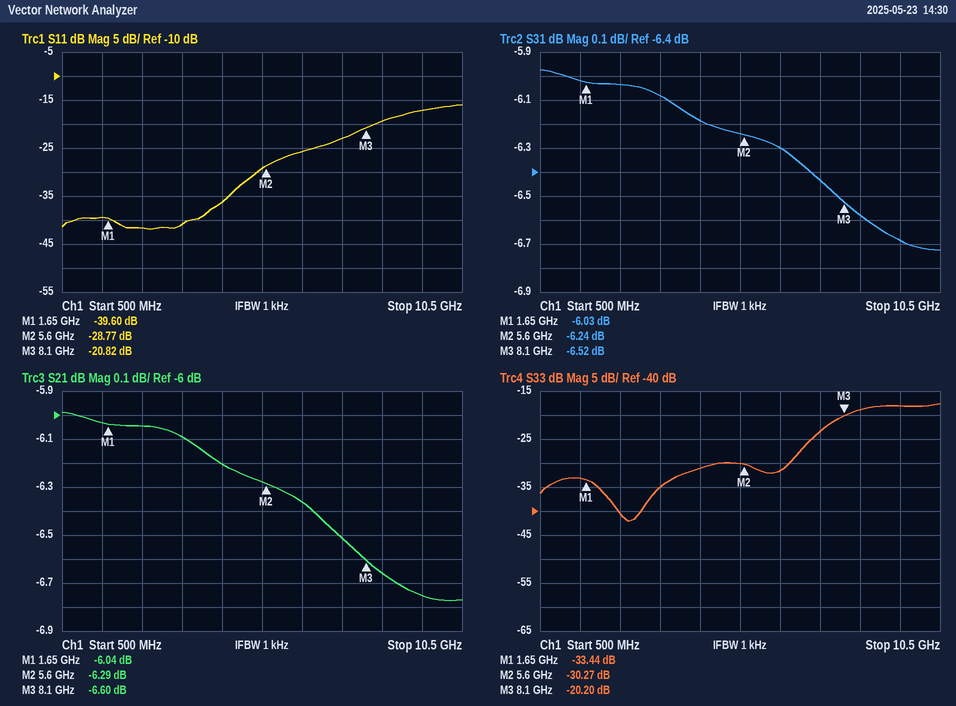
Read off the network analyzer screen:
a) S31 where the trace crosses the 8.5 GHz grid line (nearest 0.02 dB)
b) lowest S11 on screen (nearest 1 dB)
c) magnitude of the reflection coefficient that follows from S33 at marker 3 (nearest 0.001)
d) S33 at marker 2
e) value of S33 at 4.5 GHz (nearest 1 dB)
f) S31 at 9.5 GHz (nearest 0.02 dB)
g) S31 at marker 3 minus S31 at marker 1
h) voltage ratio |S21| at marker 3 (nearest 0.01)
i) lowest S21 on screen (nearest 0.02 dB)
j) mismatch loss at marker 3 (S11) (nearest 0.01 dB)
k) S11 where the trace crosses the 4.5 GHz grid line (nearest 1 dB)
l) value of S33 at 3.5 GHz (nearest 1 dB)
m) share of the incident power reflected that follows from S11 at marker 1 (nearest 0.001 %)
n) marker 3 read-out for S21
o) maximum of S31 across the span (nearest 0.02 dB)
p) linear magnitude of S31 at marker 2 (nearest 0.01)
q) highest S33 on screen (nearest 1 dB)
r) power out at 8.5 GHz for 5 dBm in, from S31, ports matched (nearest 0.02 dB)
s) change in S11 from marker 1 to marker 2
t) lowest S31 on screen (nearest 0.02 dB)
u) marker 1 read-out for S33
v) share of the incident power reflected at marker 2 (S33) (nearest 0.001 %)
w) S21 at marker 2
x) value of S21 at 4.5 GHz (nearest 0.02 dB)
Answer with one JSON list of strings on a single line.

["-6.58 dB", "-42 dB", "0.098", "-30.27 dB", "-31 dB", "-6.68 dB", "-0.49 dB", "0.47", "-6.78 dB", "0.04 dB", "-36 dB", "-35 dB", "0.011 %", "-6.60 dB", "-5.98 dB", "0.49", "-18 dB", "-1.58 dBm", "10.83 dB", "-6.72 dB", "-33.44 dB", "0.094 %", "-6.29 dB", "-6.20 dB"]
